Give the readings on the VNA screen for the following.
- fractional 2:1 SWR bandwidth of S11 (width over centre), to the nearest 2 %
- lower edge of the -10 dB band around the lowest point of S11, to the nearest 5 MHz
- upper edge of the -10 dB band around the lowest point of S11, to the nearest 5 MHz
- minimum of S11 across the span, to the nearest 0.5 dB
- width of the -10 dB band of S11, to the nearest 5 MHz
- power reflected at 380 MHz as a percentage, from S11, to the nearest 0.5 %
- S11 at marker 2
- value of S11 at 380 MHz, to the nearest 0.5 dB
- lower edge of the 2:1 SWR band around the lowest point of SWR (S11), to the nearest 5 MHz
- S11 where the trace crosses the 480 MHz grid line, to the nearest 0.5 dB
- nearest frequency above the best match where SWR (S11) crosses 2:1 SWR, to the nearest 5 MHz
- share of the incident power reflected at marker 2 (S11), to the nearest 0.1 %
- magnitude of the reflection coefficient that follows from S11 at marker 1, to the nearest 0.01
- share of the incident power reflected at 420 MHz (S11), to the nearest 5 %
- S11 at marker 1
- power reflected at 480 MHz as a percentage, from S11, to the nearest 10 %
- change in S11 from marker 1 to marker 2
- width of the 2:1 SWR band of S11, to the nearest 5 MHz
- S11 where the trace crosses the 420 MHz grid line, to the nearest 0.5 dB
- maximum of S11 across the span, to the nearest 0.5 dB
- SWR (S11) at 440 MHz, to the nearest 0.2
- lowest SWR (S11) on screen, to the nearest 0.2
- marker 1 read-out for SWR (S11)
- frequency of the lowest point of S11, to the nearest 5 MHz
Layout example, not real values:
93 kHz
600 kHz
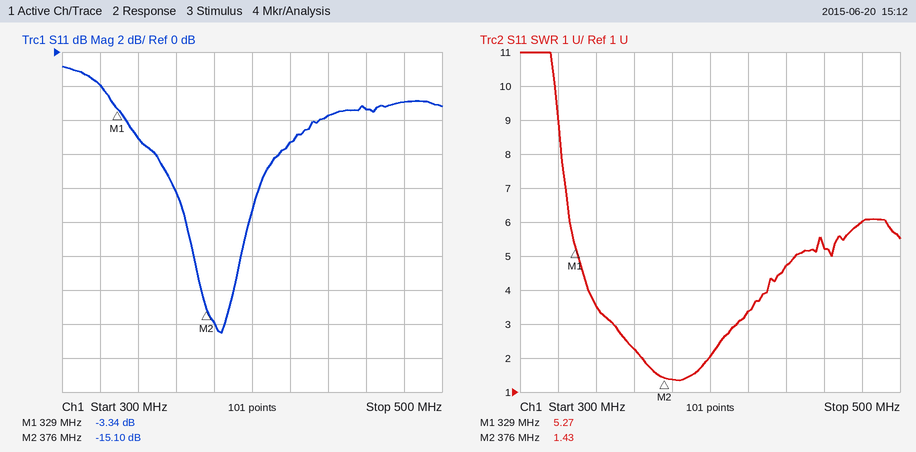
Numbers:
10 %
365 MHz
400 MHz
-16.5 dB
35 MHz
2.5 %
-15.10 dB
-16.0 dB
365 MHz
-3.0 dB
400 MHz
3.1 %
0.68
30 %
-3.34 dB
50 %
-11.76 dB
35 MHz
-5.5 dB
-1.0 dB
4.8
1.4
5.27
385 MHz
